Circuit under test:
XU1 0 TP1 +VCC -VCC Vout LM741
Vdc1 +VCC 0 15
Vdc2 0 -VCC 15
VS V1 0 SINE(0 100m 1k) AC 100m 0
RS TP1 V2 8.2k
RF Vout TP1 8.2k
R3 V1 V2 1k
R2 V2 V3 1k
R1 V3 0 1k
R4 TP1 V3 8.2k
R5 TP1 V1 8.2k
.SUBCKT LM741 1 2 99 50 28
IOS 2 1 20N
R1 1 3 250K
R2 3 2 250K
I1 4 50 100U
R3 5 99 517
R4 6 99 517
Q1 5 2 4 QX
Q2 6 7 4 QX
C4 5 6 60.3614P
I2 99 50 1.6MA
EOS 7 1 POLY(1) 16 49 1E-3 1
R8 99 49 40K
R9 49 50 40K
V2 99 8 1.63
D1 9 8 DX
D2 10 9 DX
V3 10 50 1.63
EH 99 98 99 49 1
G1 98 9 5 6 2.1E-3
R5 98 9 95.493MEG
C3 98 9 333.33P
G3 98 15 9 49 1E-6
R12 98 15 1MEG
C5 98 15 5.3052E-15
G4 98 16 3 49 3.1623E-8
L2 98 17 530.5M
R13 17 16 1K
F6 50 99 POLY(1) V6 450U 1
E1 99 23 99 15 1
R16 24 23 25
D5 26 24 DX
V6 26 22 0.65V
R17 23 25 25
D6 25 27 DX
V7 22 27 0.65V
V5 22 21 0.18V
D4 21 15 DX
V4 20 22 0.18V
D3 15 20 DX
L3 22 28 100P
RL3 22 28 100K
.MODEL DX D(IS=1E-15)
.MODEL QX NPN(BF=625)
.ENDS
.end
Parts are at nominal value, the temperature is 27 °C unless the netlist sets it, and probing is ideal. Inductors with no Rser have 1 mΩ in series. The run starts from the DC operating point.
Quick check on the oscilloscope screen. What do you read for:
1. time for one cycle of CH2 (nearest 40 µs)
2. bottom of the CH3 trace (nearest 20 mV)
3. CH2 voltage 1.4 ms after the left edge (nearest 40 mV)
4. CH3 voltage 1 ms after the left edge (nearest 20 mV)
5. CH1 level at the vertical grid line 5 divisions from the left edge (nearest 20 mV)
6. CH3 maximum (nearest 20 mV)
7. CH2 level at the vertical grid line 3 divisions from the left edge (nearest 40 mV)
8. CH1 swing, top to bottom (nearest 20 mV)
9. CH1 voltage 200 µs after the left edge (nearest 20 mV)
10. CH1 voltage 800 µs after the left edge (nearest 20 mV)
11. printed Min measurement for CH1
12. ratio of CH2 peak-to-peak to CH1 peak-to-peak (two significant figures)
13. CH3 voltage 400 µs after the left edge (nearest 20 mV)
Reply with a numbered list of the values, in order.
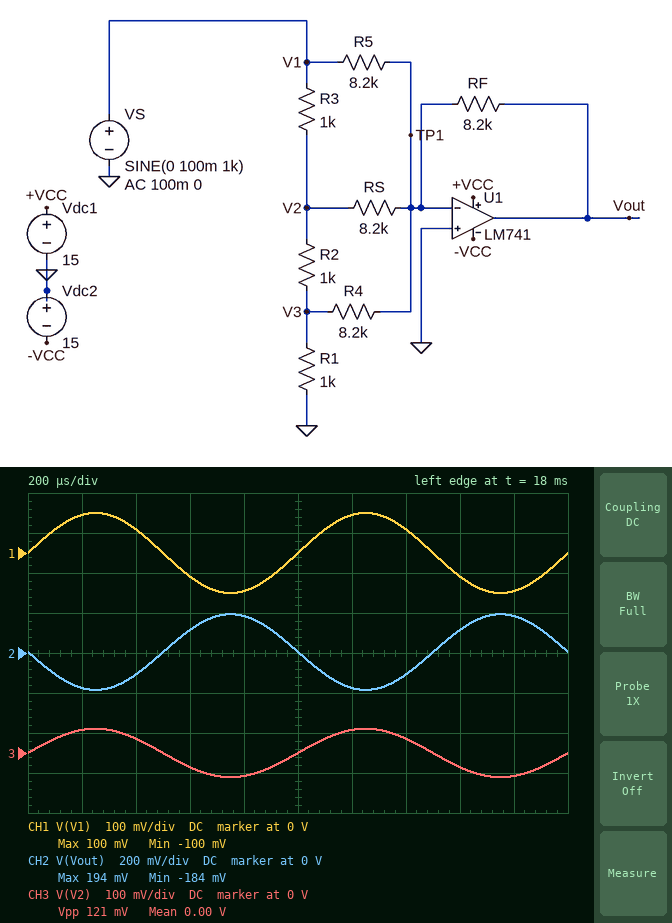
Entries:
1. 1.00 ms
2. -60 mV
3. -120 mV
4. 0 V
5. 0 V
6. 60 mV
7. 120 mV
8. 200 mV
9. 100 mV
10. -100 mV
11. -100 mV
12. 1.9
13. 40 mV
